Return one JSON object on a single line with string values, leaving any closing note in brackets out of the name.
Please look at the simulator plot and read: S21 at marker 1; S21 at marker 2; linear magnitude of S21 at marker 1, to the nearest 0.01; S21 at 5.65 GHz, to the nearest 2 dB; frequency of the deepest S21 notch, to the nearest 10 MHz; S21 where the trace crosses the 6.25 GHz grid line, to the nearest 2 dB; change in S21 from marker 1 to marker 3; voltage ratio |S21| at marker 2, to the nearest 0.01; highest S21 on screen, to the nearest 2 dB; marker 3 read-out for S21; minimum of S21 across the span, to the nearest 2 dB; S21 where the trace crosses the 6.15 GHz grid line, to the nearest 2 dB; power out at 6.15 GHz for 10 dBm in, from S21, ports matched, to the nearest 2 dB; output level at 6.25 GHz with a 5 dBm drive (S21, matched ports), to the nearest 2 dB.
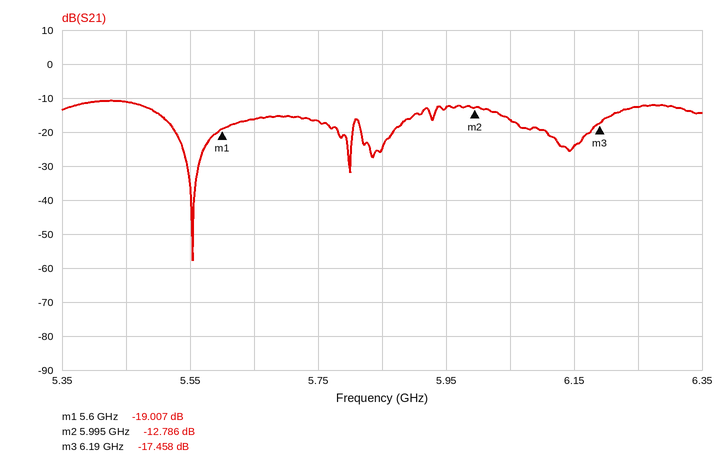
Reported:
{"S21 at marker 1": "-19.007 dB", "S21 at marker 2": "-12.786 dB", "linear magnitude of S21 at marker 1, to the nearest 0.01": "0.11", "S21 at 5.65 GHz, to the nearest 2 dB": "-16 dB", "frequency of the deepest S21 notch, to the nearest 10 MHz": "5.55 GHz", "S21 where the trace crosses the 6.25 GHz grid line, to the nearest 2 dB": "-12 dB", "change in S21 from marker 1 to marker 3": "1.549 dB", "voltage ratio |S21| at marker 2, to the nearest 0.01": "0.23", "highest S21 on screen, to the nearest 2 dB": "-10 dB", "marker 3 read-out for S21": "-17.458 dB", "minimum of S21 across the span, to the nearest 2 dB": "-58 dB", "S21 where the trace crosses the 6.15 GHz grid line, to the nearest 2 dB": "-24 dB", "power out at 6.15 GHz for 10 dBm in, from S21, ports matched, to the nearest 2 dB": "-14 dBm", "output level at 6.25 GHz with a 5 dBm drive (S21, matched ports), to the nearest 2 dB": "-8 dBm"}
